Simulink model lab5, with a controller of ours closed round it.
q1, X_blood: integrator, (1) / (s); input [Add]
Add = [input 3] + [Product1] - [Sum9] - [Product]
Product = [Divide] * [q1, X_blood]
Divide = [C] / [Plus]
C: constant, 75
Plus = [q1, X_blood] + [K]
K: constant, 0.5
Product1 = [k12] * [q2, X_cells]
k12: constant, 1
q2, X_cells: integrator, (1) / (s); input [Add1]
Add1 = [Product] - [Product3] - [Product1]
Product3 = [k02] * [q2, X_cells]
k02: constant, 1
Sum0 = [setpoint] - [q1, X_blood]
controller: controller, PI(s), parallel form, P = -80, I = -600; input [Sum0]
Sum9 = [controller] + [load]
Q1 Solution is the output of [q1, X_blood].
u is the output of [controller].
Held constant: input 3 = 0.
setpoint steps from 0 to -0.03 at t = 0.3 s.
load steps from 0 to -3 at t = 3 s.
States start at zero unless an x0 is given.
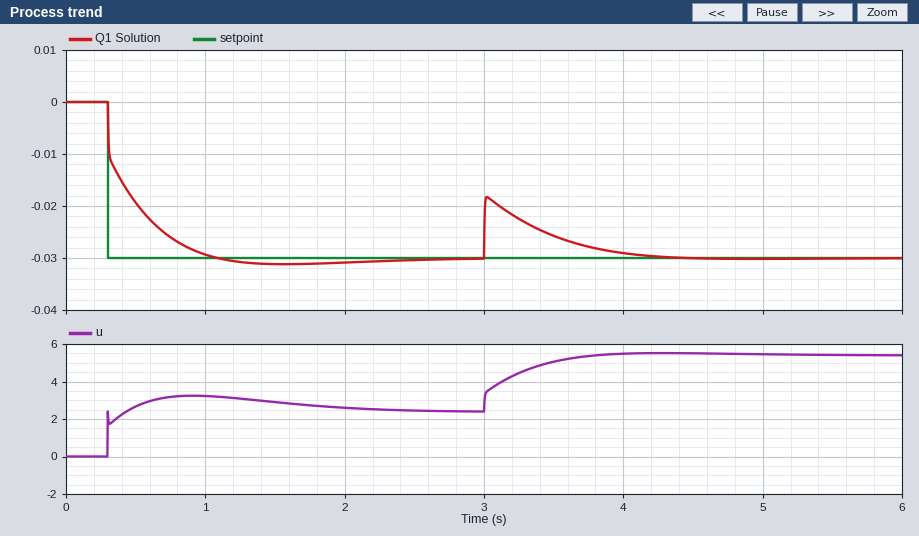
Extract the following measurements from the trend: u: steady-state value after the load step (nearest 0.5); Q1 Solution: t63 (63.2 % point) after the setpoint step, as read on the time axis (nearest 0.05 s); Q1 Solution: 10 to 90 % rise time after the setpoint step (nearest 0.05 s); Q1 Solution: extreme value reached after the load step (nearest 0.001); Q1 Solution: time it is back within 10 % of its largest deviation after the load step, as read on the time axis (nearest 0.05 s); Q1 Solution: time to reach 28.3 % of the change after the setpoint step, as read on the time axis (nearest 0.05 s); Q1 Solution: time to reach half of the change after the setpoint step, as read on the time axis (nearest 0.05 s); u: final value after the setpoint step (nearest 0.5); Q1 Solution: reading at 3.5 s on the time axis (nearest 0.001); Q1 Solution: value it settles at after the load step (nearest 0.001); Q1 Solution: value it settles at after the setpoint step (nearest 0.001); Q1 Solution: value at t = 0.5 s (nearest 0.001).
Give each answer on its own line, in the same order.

5.5
0.50 s
0.50 s
-0.018
3.95 s
0.30 s
0.40 s
2.5
-0.026
-0.030
-0.030
-0.019
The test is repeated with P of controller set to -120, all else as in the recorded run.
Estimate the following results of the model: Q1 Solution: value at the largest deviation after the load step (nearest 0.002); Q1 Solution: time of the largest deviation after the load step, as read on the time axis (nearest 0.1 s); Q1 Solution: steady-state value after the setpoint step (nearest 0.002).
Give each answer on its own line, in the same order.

-0.020
3.0 s
-0.030
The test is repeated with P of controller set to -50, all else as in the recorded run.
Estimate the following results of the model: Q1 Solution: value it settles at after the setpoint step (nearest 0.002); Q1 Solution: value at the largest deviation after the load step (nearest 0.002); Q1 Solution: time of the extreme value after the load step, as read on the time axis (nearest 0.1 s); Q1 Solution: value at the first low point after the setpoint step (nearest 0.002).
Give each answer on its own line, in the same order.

-0.030
-0.016
3.0 s
-0.032
